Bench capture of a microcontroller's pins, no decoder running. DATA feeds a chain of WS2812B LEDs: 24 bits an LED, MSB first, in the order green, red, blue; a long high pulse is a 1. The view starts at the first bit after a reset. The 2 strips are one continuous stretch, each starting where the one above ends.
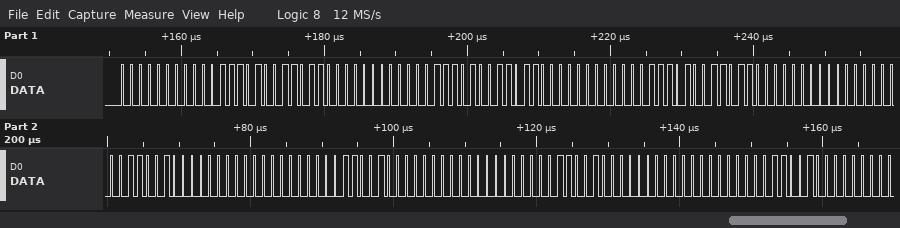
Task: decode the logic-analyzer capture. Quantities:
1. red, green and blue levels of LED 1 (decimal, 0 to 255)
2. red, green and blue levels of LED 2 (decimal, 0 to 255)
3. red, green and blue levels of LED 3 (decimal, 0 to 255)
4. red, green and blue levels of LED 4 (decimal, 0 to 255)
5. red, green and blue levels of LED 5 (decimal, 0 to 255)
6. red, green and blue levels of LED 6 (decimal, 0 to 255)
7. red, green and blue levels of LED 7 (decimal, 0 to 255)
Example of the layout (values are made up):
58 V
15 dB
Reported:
29, 0, 54
29, 0, 54
29, 0, 54
0, 0, 100
0, 0, 100
0, 0, 100
0, 0, 100
